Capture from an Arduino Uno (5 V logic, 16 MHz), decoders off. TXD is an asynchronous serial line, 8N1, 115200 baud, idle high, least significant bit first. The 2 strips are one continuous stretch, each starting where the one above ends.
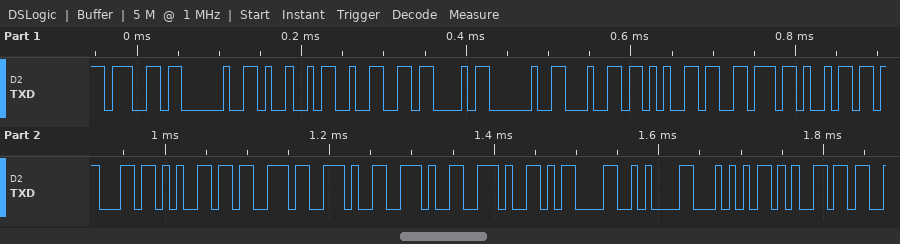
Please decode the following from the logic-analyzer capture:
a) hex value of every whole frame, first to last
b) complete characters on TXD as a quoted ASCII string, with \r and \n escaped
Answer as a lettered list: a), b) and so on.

a) 67 20 49 32 43 20 64 65 76 69 63 65 73 2E 2E 2E 0D 0A 54 65
b) "g I2C devices...\r\nTe"
